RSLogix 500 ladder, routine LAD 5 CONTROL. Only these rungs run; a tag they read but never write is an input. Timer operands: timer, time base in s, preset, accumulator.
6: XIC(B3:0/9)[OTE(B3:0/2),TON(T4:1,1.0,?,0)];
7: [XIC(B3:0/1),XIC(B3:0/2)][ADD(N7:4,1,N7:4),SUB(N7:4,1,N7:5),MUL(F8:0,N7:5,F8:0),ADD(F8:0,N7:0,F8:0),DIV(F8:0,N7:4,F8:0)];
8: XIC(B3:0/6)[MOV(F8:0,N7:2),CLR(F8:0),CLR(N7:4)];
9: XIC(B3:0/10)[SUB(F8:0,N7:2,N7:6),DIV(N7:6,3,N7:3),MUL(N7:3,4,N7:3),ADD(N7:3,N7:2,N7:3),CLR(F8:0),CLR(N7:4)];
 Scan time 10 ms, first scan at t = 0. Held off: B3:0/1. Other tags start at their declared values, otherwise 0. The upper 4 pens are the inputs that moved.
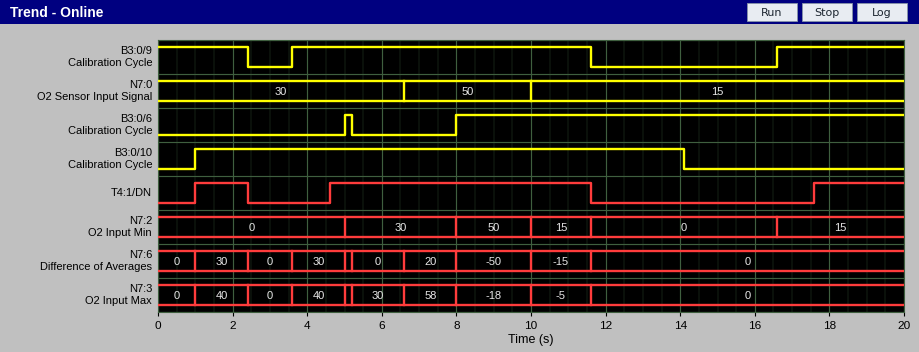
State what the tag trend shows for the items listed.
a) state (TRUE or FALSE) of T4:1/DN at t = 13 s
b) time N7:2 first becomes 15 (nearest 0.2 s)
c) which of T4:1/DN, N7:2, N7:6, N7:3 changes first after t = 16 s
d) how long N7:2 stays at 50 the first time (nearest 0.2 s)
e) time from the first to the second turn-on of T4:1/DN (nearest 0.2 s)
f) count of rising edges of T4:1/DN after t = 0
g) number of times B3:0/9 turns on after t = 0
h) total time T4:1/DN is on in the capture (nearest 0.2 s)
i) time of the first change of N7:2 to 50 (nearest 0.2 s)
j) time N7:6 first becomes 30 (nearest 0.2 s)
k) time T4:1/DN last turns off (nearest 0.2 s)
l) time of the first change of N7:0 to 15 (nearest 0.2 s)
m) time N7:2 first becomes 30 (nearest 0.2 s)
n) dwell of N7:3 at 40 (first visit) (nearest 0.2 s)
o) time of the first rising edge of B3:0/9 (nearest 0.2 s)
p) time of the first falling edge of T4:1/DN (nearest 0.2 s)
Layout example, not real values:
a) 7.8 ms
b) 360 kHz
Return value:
a) FALSE
b) 10.0 s
c) N7:2
d) 2.0 s
e) 3.6 s
f) 3
g) 2
h) 10.8 s
i) 8.0 s
j) 1.0 s
k) 11.6 s
l) 10.0 s
m) 5.0 s
n) 1.4 s
o) 3.6 s
p) 2.4 s
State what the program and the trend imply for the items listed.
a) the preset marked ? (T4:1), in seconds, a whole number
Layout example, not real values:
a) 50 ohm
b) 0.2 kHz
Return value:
a) 1 s
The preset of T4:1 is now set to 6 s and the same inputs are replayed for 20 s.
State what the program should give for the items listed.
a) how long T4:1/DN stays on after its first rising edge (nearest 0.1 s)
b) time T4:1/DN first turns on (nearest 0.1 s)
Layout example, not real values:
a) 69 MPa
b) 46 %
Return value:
a) 2.0 s
b) 9.6 s
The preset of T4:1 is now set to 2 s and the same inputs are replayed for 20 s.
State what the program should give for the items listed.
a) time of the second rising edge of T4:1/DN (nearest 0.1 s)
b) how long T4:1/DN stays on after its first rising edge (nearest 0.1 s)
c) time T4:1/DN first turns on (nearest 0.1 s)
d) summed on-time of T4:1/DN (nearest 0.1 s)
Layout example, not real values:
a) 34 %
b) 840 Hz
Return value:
a) 5.6 s
b) 0.4 s
c) 2.0 s
d) 7.8 s
